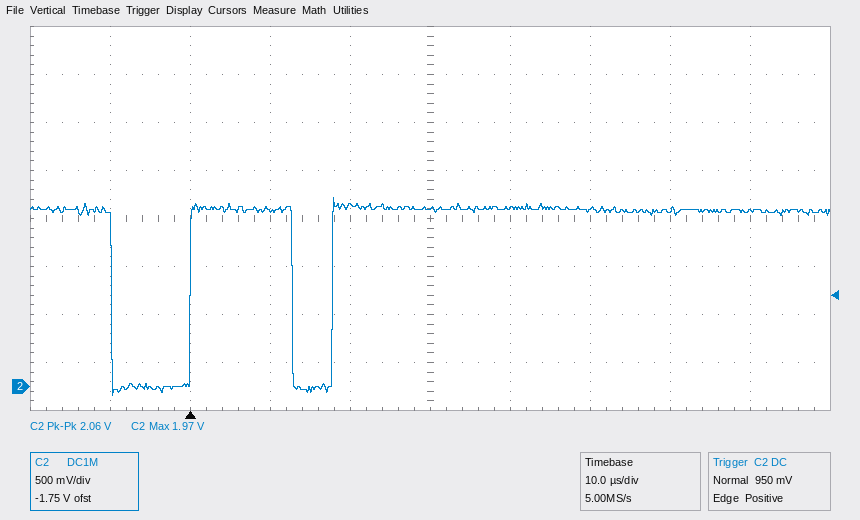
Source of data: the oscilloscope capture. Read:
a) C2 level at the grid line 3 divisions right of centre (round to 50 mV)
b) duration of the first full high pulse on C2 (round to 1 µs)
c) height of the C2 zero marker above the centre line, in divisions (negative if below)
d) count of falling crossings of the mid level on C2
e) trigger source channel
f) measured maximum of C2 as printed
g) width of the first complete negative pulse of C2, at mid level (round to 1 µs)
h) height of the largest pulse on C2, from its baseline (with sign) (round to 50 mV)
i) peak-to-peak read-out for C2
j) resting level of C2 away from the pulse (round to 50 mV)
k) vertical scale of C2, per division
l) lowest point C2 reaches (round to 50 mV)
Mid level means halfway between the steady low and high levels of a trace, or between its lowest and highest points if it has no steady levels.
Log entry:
1.85 V
13 µs
-3.5 div
2
C2
1.97 V
10 µs
-1.95 V
2.06 V
1.85 V
500 mV
-100 mV
